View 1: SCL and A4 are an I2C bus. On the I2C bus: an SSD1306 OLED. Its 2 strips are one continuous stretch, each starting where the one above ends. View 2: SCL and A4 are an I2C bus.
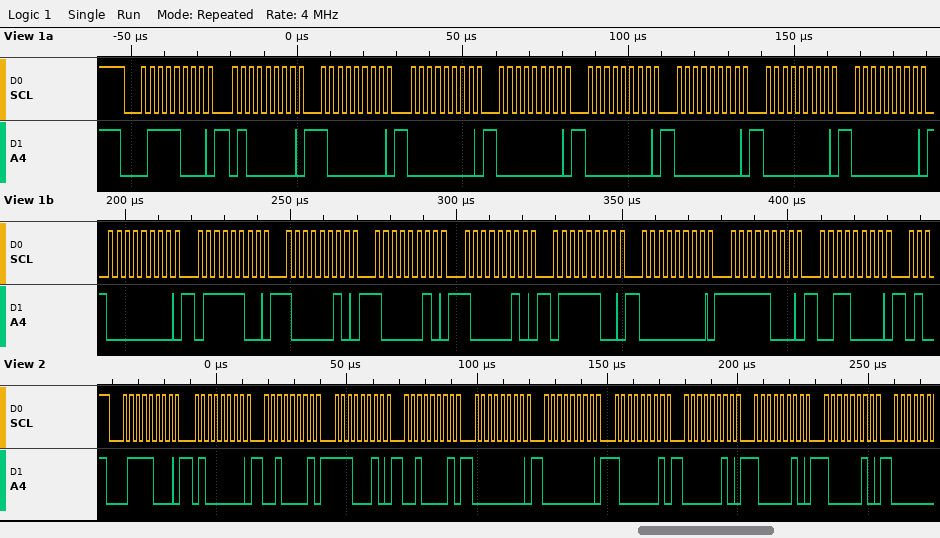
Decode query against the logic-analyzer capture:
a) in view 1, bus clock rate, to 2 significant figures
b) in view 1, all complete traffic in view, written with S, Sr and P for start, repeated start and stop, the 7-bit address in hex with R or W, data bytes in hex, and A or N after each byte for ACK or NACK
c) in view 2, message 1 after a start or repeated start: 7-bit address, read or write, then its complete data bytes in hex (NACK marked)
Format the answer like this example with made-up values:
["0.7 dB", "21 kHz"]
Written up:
["400 kHz", "S 3CW A 40 A 80 A 00 A 00 A 00 A 00 A 00 A 00 A 00 A 7C A 82 A 82 A 82 A 7C A 00 A F8 A 30 A", "0x3C write: 40 21 E2 21 00 00 81 02 82 82"]
